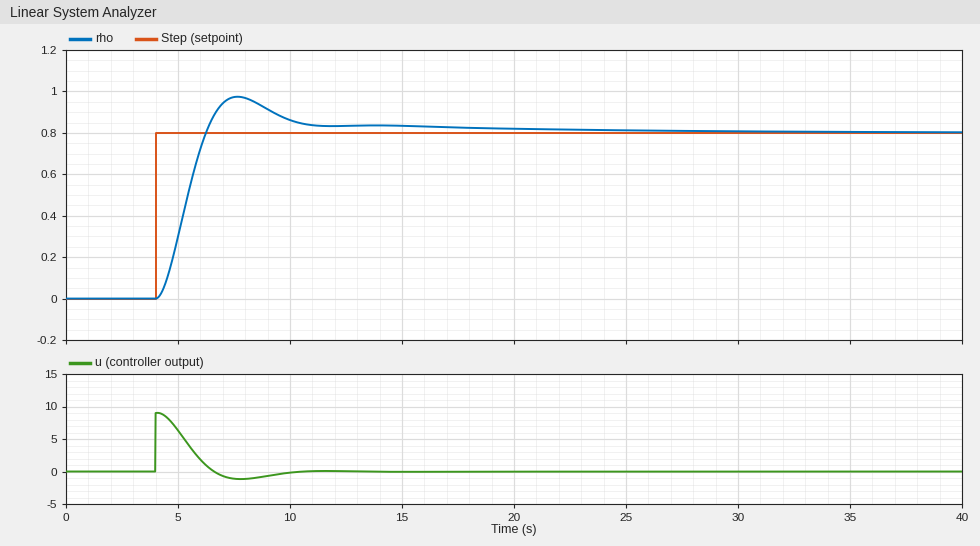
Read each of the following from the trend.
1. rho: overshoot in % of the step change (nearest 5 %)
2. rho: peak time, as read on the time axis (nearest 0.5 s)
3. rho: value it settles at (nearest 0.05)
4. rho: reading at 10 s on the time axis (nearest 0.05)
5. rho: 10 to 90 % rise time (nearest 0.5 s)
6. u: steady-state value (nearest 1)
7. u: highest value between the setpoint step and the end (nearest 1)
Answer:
20 %
7.5 s
0.80
0.85
1.5 s
0
9
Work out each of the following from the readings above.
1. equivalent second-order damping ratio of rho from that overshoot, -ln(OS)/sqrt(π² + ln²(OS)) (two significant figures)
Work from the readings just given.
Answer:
0.46
